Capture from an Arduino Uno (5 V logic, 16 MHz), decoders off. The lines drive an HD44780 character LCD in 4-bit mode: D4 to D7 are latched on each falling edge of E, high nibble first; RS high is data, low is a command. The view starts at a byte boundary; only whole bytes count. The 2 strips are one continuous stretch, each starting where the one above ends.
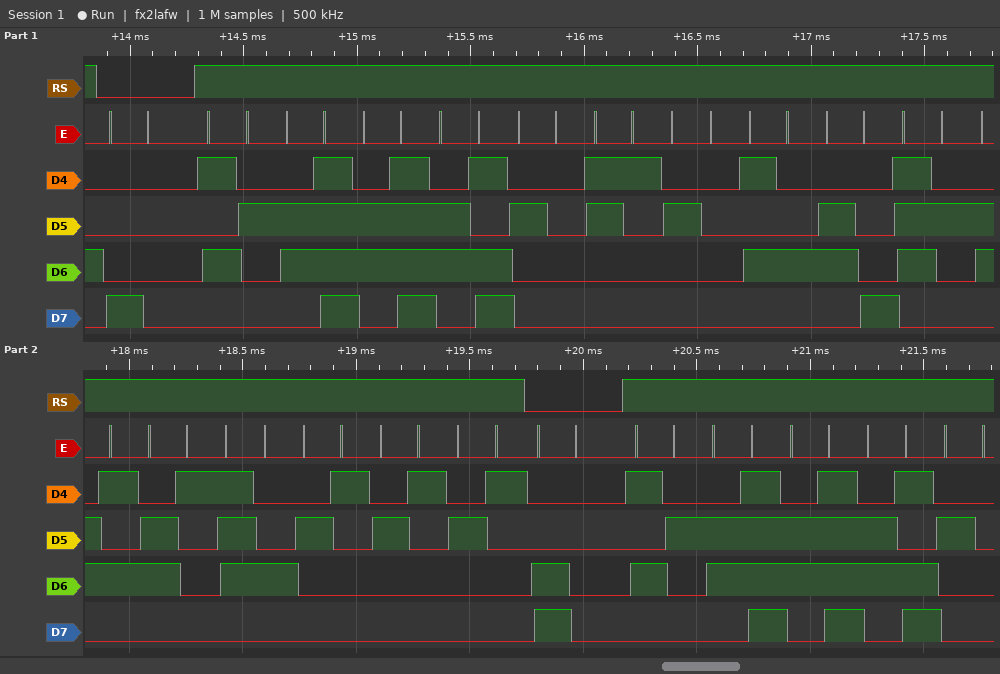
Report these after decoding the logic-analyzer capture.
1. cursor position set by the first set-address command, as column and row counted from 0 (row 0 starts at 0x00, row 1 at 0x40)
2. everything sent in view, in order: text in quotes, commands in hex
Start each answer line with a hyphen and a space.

- column 0, row 0
- 0x80 "Room 1 Threat!!!" 0xC0 "Room "
